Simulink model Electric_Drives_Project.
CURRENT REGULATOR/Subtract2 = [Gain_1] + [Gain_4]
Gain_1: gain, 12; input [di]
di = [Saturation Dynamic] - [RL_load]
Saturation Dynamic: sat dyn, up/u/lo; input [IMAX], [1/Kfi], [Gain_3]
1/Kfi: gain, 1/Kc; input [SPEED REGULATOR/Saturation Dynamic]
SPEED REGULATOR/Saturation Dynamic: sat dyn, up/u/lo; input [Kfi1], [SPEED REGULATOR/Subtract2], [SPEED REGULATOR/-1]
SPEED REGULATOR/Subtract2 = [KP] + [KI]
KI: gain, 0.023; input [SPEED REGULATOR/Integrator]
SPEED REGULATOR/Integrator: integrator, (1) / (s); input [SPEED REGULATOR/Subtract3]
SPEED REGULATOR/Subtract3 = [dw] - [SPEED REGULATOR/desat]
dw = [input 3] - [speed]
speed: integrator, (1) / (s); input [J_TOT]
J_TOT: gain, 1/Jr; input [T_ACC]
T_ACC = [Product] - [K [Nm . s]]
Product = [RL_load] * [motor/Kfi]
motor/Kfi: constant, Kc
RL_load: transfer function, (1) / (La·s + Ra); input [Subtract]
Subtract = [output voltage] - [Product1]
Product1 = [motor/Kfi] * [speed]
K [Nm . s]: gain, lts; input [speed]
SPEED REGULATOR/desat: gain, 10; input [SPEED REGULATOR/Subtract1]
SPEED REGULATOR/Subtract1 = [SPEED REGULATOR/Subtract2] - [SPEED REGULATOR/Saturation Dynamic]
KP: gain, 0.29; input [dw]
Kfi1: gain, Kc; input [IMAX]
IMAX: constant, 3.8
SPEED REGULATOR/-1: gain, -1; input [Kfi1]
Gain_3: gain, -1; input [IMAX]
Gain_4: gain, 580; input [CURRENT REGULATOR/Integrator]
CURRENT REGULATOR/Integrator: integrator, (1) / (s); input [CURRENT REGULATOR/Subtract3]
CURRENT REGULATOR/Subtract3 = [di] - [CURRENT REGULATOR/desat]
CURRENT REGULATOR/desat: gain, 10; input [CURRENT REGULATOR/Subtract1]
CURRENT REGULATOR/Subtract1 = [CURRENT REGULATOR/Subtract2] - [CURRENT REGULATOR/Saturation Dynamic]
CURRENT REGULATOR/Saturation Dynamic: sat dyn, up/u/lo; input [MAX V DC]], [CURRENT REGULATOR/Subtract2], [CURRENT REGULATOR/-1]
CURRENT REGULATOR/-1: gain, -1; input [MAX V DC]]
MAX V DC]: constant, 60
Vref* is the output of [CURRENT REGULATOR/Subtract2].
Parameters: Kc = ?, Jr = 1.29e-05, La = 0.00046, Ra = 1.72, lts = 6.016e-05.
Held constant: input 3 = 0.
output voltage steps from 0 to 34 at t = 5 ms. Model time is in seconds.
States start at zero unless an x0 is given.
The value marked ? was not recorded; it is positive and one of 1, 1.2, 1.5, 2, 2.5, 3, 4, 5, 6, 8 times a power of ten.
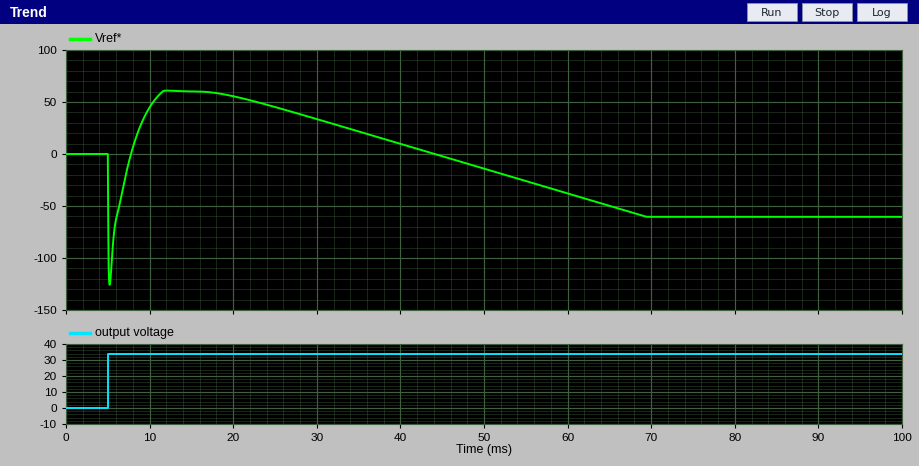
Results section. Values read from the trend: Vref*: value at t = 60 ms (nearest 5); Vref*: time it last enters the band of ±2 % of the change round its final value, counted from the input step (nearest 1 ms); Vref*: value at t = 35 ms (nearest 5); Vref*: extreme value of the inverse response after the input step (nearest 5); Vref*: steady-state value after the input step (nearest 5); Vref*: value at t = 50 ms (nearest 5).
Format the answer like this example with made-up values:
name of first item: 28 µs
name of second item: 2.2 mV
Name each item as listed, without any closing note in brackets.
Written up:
Vref*: value at t = 60 ms: -40
Vref*: time it last enters the band of ±2 % of the change round its final value, counted from the input step: 64 ms
Vref*: value at t = 35 ms: 20
Vref*: extreme value of the inverse response after the input step: 60
Vref*: steady-state value after the input step: -60
Vref*: value at t = 50 ms: -15
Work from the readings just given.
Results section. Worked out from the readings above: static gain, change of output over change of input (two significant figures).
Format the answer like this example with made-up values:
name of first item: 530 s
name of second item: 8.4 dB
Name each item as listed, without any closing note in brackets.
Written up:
static gain, change of output over change of input: -1.8
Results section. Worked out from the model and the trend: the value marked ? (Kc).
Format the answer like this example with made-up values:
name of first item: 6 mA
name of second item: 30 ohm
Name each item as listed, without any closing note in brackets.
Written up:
the value marked ?: 0.08
